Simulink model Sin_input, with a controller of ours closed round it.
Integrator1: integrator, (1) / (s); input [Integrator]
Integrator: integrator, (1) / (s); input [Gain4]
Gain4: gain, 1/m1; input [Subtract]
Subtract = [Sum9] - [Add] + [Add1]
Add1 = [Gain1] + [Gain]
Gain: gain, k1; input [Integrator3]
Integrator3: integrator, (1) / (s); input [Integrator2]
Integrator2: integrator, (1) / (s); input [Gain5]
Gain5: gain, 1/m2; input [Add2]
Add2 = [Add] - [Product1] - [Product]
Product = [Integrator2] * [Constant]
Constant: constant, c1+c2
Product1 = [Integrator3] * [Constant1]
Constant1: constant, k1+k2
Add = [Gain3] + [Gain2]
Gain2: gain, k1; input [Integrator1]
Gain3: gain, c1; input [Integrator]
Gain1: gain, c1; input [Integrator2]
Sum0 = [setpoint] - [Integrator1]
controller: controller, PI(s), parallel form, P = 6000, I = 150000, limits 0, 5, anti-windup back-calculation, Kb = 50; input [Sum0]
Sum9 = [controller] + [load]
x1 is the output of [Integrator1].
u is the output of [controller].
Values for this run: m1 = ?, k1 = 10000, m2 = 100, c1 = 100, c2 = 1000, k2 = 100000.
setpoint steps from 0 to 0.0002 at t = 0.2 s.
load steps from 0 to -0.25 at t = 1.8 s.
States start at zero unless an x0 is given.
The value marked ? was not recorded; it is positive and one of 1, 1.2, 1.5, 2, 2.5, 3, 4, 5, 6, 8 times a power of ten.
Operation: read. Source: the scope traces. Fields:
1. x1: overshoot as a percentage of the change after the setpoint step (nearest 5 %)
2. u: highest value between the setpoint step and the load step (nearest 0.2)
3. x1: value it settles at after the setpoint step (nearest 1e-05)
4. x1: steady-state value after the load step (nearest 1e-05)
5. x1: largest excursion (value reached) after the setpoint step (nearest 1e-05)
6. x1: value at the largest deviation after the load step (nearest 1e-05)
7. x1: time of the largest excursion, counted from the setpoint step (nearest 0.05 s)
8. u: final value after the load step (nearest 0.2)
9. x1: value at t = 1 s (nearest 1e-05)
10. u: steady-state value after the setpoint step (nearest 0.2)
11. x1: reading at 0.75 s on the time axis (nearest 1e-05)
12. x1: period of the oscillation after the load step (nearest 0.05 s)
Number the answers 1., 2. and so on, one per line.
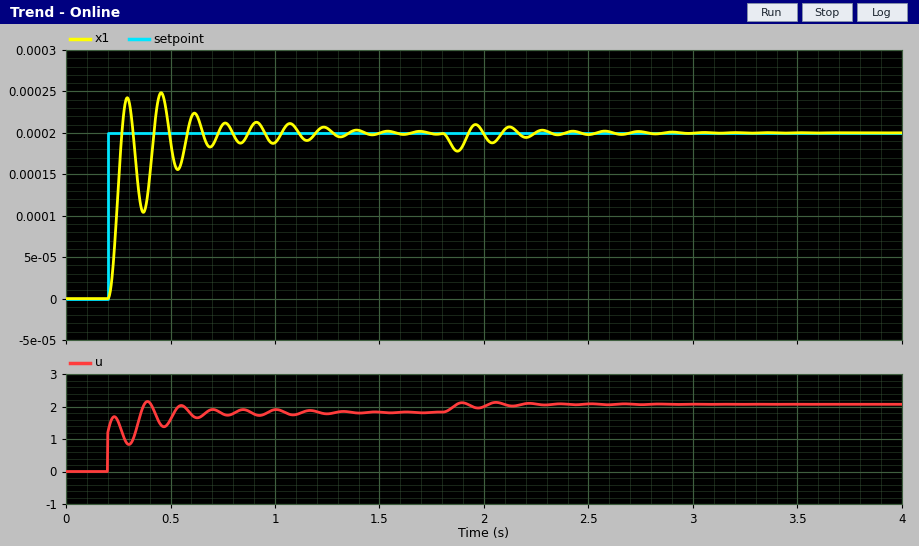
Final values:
1. 25 %
2. 2.2
3. 0.00020
4. 0.00020
5. 0.00025
6. 0.00018
7. 0.25 s
8. 2.0
9. 0.00019
10. 1.8
11. 0.00021
12. 0.15 s
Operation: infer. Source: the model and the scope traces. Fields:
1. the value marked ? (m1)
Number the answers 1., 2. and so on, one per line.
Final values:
1. 10
